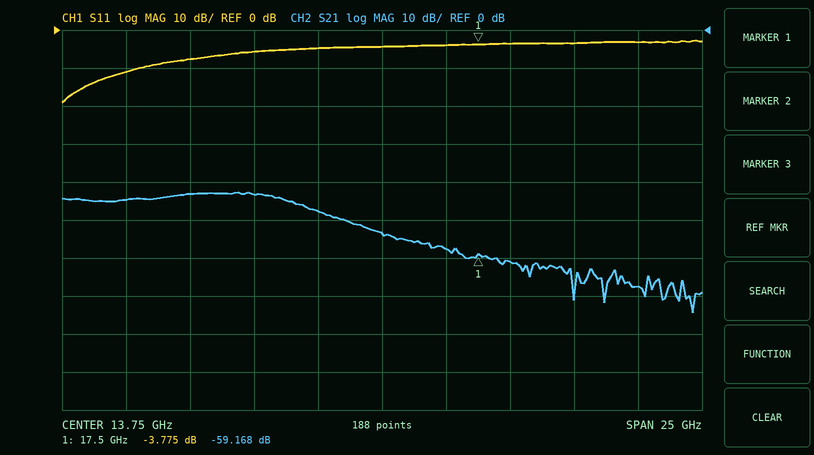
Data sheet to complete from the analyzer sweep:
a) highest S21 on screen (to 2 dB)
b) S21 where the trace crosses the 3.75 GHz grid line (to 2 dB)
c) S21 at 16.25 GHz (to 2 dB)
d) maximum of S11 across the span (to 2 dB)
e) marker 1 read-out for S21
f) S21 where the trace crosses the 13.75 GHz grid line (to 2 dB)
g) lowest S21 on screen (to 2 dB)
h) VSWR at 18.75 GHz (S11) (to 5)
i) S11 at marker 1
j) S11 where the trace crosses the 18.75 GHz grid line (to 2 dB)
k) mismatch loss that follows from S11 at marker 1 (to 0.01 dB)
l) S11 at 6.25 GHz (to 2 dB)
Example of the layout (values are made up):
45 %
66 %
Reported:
-42 dB
-44 dB
-58 dB
-2 dB
-59.168 dB
-54 dB
-74 dB
5
-3.775 dB
-4 dB
2.36 dB
-8 dB
